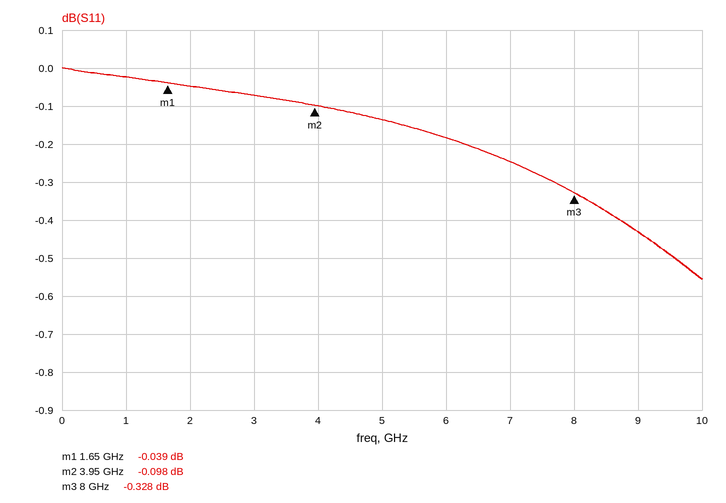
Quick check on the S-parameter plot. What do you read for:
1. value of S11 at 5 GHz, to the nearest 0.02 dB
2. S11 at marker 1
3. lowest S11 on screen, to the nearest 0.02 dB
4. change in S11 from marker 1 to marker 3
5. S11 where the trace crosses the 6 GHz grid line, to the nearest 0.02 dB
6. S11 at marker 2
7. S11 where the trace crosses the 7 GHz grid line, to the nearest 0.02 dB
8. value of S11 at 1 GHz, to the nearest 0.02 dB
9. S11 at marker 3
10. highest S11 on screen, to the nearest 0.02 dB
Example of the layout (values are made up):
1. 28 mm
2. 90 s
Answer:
1. -0.14 dB
2. -0.039 dB
3. -0.56 dB
4. -0.289 dB
5. -0.18 dB
6. -0.098 dB
7. -0.24 dB
8. -0.02 dB
9. -0.328 dB
10. 0.00 dB
